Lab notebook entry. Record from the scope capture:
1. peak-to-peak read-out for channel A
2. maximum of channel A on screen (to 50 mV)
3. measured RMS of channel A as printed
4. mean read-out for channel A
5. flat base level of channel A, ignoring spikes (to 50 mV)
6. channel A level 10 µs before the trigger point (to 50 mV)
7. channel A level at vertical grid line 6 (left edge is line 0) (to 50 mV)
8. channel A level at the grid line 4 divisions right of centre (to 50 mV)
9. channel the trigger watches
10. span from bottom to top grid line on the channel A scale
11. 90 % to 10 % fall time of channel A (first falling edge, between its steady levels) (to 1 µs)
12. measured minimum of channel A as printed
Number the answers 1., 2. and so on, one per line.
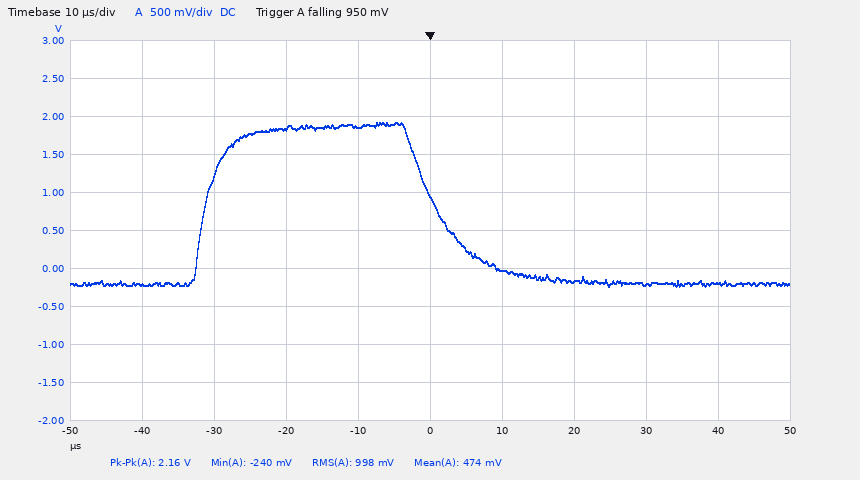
1. 2.16 V
2. 1.90 V
3. 998 mV
4. 474 mV
5. -200 mV
6. 1.85 V
7. 0 mV
8. -200 mV
9. channel A
10. 5 V
11. 12 µs
12. -240 mV
